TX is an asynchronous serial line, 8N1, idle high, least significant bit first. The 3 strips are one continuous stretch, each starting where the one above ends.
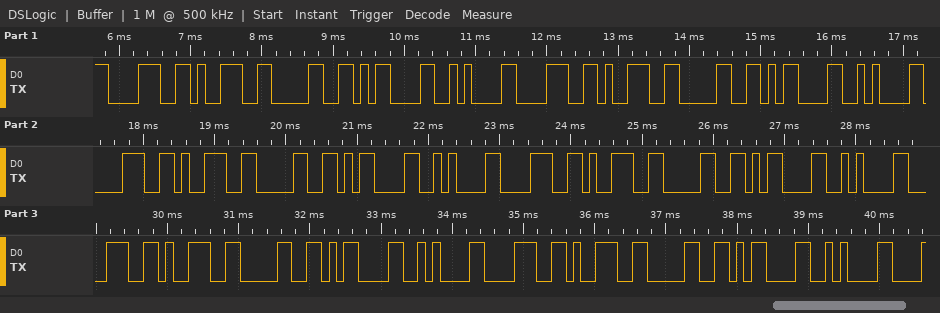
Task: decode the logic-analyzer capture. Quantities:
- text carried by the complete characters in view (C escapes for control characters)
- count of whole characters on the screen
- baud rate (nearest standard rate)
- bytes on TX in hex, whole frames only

"890\r\n890\r\n890\r\n890\r\n890\r\n890\r\n"
30
9600 baud
38 39 30 0D 0A 38 39 30 0D 0A 38 39 30 0D 0A 38 39 30 0D 0A 38 39 30 0D 0A 38 39 30 0D 0A
